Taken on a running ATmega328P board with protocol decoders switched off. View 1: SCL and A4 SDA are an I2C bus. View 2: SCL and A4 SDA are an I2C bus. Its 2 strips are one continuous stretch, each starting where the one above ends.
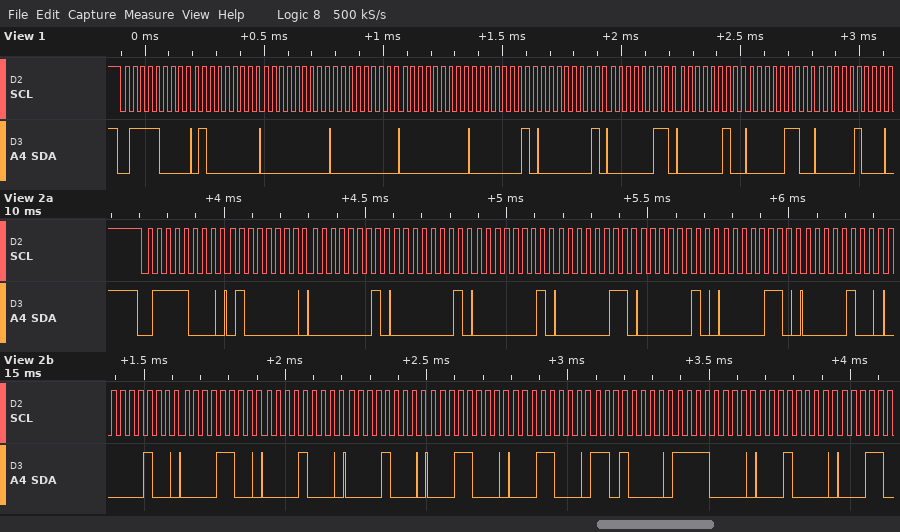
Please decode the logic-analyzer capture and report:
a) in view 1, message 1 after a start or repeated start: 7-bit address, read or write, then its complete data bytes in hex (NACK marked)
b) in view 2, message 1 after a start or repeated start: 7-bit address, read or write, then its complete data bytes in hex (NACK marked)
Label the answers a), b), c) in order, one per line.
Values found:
a) 0x3C write: 40 00 00 00 01 01 03 02 06 04
b) 0x3C write: 40 01 01 01 03 02 06 04 04 0C 08 08 18 18 D0 F0 10
